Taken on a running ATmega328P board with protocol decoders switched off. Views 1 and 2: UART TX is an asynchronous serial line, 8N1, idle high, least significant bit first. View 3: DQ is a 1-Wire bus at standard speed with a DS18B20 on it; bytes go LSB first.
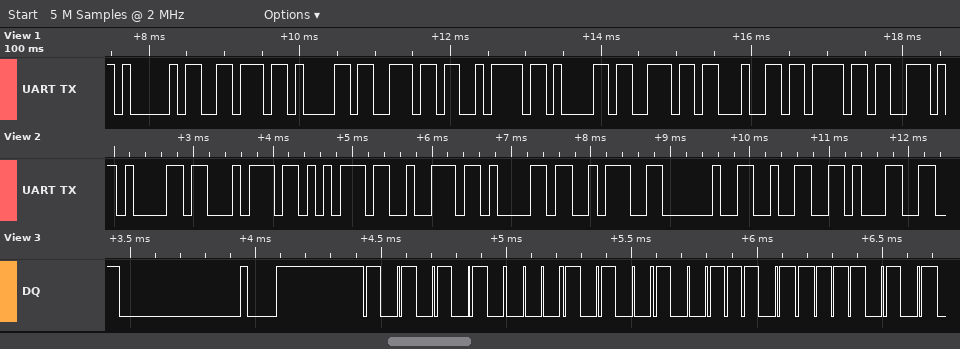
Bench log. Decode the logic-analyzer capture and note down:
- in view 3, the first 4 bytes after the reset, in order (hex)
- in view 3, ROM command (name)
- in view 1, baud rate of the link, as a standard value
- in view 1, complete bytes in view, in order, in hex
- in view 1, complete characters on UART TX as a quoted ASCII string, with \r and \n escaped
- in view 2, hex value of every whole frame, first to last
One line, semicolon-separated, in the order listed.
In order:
55 28 B9 AF; Match ROM; 9600 baud; 41 76 61 6E 7A 61 6E 64 6F; "Avanzando"; 61 74 75 72 61 3A 20 32 31
